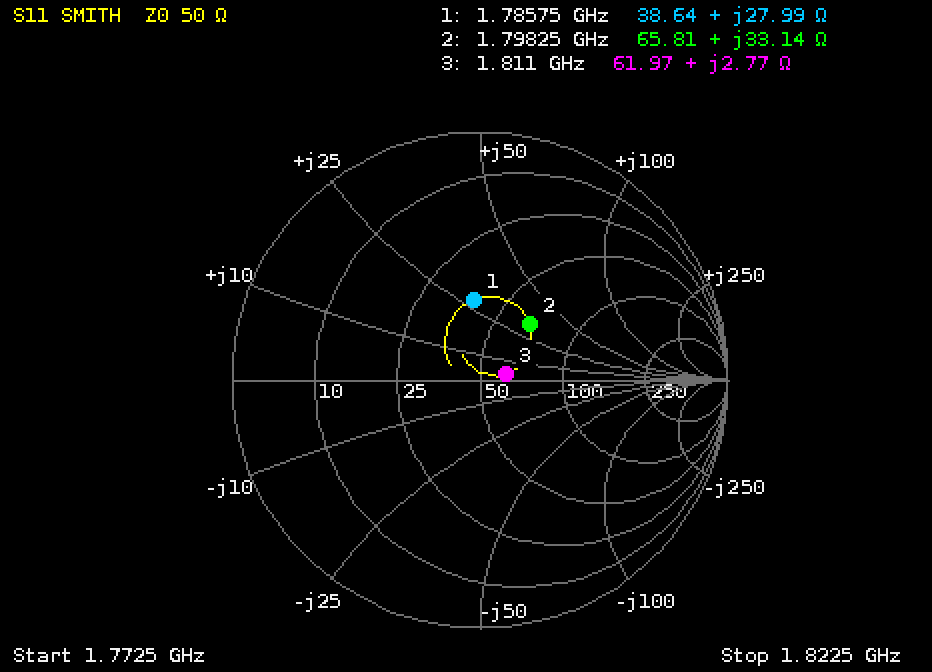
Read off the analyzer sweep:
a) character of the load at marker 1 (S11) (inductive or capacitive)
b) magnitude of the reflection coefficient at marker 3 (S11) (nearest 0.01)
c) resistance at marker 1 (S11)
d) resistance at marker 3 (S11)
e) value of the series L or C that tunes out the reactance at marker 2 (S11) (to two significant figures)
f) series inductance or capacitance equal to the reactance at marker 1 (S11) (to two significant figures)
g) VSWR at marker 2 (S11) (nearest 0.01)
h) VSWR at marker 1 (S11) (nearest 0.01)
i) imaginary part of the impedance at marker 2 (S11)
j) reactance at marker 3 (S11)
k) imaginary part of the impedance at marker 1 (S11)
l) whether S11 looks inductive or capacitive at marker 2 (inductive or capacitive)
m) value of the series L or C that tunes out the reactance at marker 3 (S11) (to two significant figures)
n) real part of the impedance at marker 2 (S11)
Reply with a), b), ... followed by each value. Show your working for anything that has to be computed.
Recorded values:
a) inductive
b) 0.11
c) 38.64 Ω
d) 61.97 Ω
e) C = 1/(2π × 1.79825 GHz × 33.14 Ω) ≈ 2.7 pF
f) L = 27.99 Ω/(2π × 1.78575 GHz) ≈ 2.5 nH
g) 1.88
h) 1.96
i) +33.14 Ω
j) +2.77 Ω
k) +27.99 Ω
l) inductive
m) C = 1/(2π × 1.811 GHz × 2.77 Ω) ≈ 32 pF
n) 65.81 Ω
